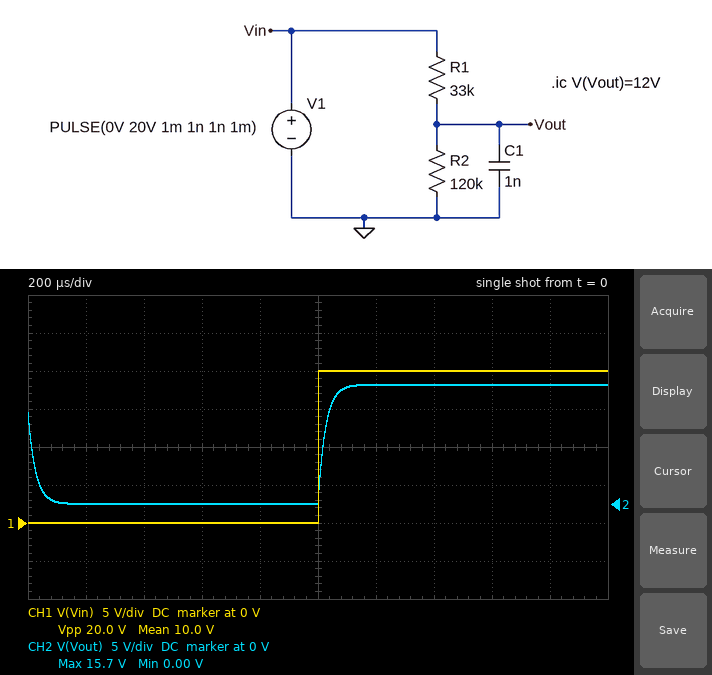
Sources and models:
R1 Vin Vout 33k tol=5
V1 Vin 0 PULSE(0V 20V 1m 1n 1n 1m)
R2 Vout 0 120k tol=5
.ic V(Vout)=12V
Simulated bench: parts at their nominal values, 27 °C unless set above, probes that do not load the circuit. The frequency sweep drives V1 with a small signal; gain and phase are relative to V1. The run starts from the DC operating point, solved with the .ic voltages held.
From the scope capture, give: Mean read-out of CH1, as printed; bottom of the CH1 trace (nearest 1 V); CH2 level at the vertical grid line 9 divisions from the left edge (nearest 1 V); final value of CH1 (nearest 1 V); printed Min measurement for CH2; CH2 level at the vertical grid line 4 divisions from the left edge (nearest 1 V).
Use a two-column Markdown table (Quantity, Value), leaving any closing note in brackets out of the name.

| Quantity | Value |
|---|---|
| Mean read-out of CH1, as printed | 10.0 V |
| bottom of the CH1 trace | 0 V |
| CH2 level at the vertical grid line 9 divisions from the left edge | 16 V |
| final value of CH1 | 20 V |
| printed Min measurement for CH2 | 0.00 V |
| CH2 level at the vertical grid line 4 divisions from the left edge | 0 V |
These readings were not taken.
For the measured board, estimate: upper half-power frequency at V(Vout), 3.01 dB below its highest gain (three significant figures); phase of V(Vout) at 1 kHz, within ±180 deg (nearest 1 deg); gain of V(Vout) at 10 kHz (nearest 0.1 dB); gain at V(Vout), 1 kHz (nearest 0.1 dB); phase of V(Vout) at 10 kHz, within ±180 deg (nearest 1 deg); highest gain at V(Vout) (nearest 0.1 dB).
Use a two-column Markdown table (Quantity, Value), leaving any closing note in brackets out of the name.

| Quantity | Value |
|---|---|
| upper half-power frequency at V(Vout), 3.01 dB below its highest gain | 6.15 kHz |
| phase of V(Vout) at 1 kHz, within ±180 deg | -9 deg |
| gain of V(Vout) at 10 kHz | -7.7 dB |
| gain at V(Vout), 1 kHz | -2.2 dB |
| phase of V(Vout) at 10 kHz, within ±180 deg | -58 deg |
| highest gain at V(Vout) | -2.1 dB |
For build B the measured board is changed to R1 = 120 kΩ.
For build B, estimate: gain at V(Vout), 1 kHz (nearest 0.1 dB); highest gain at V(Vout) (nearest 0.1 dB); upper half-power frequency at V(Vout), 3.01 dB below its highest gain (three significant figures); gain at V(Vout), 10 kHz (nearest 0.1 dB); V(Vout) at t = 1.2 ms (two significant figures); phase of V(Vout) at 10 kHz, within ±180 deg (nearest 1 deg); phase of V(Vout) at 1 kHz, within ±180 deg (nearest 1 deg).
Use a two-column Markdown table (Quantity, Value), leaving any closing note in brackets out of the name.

| Quantity | Value |
|---|---|
| gain at V(Vout), 1 kHz | -6.6 dB |
| highest gain at V(Vout) | -6.0 dB |
| upper half-power frequency at V(Vout), 3.01 dB below its highest gain | 2.65 kHz |
| gain at V(Vout), 10 kHz | -17.8 dB |
| V(Vout) at t = 1.2 ms | 9.6 V |
| phase of V(Vout) at 10 kHz, within ±180 deg | -75 deg |
| phase of V(Vout) at 1 kHz, within ±180 deg | -21 deg |
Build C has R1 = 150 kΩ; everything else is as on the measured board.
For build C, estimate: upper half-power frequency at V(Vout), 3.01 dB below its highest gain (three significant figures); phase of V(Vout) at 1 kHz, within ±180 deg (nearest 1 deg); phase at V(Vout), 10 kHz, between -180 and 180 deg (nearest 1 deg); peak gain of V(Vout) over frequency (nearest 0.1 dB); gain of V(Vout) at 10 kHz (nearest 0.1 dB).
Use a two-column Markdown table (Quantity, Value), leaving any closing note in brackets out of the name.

| Quantity | Value |
|---|---|
| upper half-power frequency at V(Vout), 3.01 dB below its highest gain | 2.39 kHz |
| phase of V(Vout) at 1 kHz, within ±180 deg | -23 deg |
| phase at V(Vout), 10 kHz, between -180 and 180 deg | -77 deg |
| peak gain of V(Vout) over frequency | -7.0 dB |
| gain of V(Vout) at 10 kHz | -19.7 dB |
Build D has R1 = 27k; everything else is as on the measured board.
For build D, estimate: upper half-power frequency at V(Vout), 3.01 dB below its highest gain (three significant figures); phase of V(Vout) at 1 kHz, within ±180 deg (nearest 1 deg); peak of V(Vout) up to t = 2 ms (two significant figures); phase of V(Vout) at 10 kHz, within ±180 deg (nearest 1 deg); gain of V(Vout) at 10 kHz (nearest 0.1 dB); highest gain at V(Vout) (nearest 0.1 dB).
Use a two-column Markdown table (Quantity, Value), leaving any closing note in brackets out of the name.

| Quantity | Value |
|---|---|
| upper half-power frequency at V(Vout), 3.01 dB below its highest gain | 7.22 kHz |
| phase of V(Vout) at 1 kHz, within ±180 deg | -8 deg |
| peak of V(Vout) up to t = 2 ms | 16 V |
| phase of V(Vout) at 10 kHz, within ±180 deg | -54 deg |
| gain of V(Vout) at 10 kHz | -6.4 dB |
| highest gain at V(Vout) | -1.8 dB |
